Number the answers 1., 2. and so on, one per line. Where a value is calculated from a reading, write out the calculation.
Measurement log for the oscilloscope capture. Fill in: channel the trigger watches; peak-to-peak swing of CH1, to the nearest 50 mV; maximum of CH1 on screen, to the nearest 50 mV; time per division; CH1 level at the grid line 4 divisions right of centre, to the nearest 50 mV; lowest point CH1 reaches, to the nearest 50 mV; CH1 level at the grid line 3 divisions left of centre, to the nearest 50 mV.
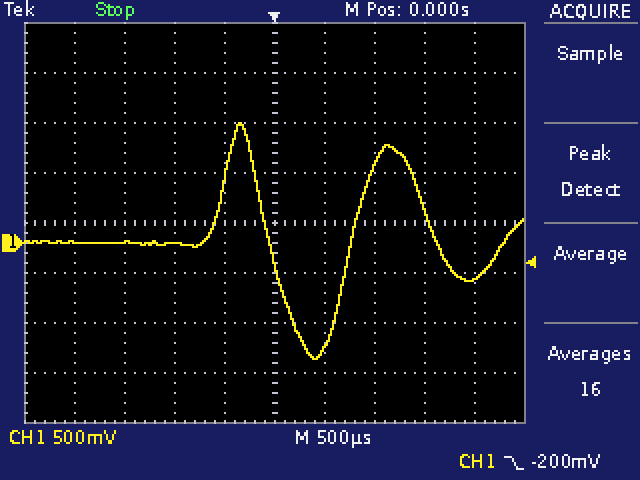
1. CH1
2. 1.20 V − (-1.15 V) = 2.35 V
3. 1.20 V
4. 500 µs
5. -350 mV
6. -1.15 V
7. 0 mV
